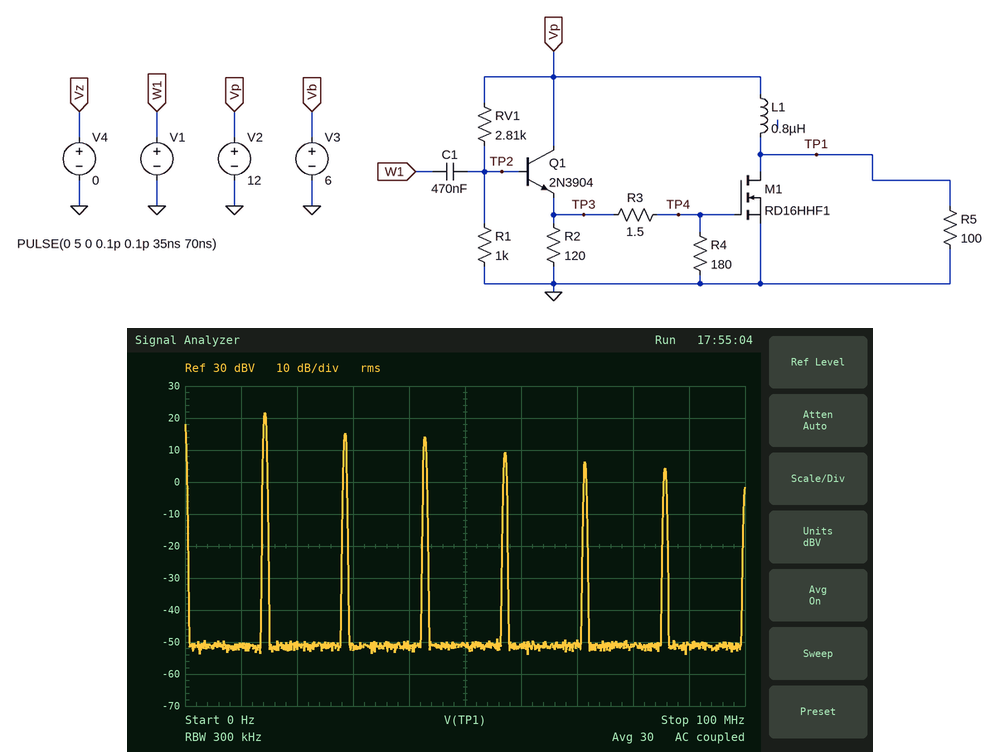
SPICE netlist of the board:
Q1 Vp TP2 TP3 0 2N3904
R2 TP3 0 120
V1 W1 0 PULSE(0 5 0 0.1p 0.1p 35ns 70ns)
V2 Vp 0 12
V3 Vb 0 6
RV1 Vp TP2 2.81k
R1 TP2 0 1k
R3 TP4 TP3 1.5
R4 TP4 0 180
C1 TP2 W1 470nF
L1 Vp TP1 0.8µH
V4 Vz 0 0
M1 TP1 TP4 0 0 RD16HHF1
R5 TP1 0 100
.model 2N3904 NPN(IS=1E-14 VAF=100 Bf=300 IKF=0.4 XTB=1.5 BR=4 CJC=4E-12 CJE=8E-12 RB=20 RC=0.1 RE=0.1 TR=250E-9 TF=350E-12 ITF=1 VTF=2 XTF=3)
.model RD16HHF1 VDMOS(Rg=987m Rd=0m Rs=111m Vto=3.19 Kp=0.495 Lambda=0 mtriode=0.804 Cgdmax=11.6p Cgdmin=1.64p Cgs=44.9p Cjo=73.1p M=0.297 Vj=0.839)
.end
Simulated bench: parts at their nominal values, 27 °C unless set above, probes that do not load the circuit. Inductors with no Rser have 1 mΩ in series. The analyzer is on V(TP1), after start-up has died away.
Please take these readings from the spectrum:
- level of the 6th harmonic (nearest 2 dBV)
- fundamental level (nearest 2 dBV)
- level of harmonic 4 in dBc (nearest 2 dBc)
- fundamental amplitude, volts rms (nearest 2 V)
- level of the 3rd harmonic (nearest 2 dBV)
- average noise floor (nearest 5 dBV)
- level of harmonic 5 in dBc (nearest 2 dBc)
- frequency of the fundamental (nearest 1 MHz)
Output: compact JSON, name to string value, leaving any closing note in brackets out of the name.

{"level of the 6th harmonic": "4 dBV", "fundamental level": "22 dBV", "level of harmonic 4 in dBc": "-12 dBc", "fundamental amplitude, volts rms": "12 V", "level of the 3rd harmonic": "14 dBV", "average noise floor": "-50 dBV", "level of harmonic 5 in dBc": "-16 dBc", "frequency of the fundamental": "14 MHz"}
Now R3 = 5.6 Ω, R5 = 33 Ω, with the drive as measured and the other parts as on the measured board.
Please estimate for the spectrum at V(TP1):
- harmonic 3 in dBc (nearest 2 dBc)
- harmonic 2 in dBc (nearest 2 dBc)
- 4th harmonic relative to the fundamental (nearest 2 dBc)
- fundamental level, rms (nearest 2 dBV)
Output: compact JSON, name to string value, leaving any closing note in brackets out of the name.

{"harmonic 3 in dBc": "-10 dBc", "harmonic 2 in dBc": "-14 dBc", "4th harmonic relative to the fundamental": "-18 dBc", "fundamental level, rms": "20 dBV"}
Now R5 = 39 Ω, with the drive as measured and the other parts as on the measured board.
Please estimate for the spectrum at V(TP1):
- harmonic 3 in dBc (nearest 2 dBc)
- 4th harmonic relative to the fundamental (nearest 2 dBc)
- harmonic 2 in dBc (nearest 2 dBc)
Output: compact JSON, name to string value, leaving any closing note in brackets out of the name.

{"harmonic 3 in dBc": "-10 dBc", "4th harmonic relative to the fundamental": "-18 dBc", "harmonic 2 in dBc": "-14 dBc"}
